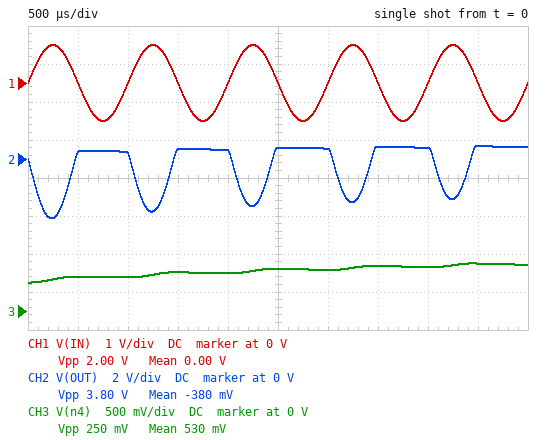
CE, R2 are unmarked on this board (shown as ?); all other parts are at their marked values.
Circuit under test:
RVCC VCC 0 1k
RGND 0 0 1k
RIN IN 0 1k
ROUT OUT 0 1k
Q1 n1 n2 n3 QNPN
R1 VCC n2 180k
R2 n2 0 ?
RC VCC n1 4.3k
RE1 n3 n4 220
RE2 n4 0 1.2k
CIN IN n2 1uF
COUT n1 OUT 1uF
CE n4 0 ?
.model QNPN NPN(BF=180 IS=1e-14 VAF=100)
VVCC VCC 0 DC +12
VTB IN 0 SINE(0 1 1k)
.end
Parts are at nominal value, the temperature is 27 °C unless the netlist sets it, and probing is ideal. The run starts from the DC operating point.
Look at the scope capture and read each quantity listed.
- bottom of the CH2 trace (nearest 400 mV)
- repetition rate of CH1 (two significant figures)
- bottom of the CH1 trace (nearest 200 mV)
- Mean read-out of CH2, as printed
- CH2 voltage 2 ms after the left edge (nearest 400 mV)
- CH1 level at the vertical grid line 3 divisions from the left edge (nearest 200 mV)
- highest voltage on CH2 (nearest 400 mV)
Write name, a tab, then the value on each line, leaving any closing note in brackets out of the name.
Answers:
bottom of the CH2 trace	-3.2 V
repetition rate of CH1	1.0 kHz
bottom of the CH1 trace	-1.0 V
Mean read-out of CH2, as printed	-380 mV
CH2 voltage 2 ms after the left edge	400 mV
CH1 level at the vertical grid line 3 divisions from the left edge	0 V
highest voltage on CH2	800 mV
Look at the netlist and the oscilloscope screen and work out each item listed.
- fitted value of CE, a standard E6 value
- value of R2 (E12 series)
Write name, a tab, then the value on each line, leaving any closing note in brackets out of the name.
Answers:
fitted value of CE, a standard E6 value	15 µF
value of R2	18 kΩ
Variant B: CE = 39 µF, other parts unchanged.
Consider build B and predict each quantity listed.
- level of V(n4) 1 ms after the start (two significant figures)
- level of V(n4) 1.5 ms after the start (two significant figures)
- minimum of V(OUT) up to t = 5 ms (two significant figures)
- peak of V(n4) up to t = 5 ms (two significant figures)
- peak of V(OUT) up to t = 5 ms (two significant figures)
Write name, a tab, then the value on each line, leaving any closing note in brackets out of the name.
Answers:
level of V(n4) 1 ms after the start	400 mV
level of V(n4) 1.5 ms after the start	430 mV
minimum of V(OUT) up to t = 5 ms	-3.2 V
peak of V(n4) up to t = 5 ms	500 mV
peak of V(OUT) up to t = 5 ms	760 mV
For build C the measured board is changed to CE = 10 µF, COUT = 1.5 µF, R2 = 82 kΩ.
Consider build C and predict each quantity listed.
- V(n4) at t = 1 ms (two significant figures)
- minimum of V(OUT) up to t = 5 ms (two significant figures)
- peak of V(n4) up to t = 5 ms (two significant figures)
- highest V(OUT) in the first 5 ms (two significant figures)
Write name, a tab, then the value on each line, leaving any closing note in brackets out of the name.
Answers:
V(n4) at t = 1 ms	2.1 V
minimum of V(OUT) up to t = 5 ms	-2.1 V
peak of V(n4) up to t = 5 ms	2.2 V
highest V(OUT) in the first 5 ms	1.5 V
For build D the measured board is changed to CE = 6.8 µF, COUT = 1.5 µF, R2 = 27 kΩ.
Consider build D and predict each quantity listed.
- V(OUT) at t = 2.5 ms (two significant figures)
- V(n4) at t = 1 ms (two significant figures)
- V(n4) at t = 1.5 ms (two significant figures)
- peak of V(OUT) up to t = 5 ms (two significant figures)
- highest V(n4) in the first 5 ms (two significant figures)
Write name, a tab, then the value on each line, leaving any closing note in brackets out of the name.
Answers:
V(OUT) at t = 2.5 ms	680 mV
V(n4) at t = 1 ms	830 mV
V(n4) at t = 1.5 ms	960 mV
peak of V(OUT) up to t = 5 ms	720 mV
highest V(n4) in the first 5 ms	1.1 V
